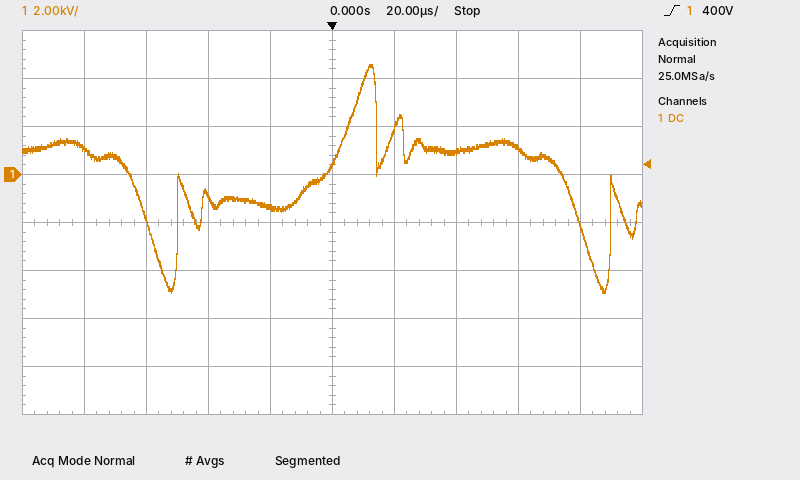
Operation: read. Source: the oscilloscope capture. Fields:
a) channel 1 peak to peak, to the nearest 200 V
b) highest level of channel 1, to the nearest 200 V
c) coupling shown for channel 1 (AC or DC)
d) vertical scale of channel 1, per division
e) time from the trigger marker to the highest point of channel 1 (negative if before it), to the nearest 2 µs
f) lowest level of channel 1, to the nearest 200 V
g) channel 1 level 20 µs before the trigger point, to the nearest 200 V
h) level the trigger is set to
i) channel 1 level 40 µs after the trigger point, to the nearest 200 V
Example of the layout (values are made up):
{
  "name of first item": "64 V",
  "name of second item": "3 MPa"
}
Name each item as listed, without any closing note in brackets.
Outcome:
{
  "channel 1 peak to peak, to the nearest 200 V": "9.6 kV",
  "highest level of channel 1, to the nearest 200 V": "4.6 kV",
  "coupling shown for channel 1": "DC",
  "vertical scale of channel 1, per division": "2 kV",
  "time from the trigger marker to the highest point of channel 1 (negative if before it), to the nearest 2 µs": "+12 µs",
  "lowest level of channel 1, to the nearest 200 V": "-5.0 kV",
  "channel 1 level 20 µs before the trigger point, to the nearest 200 V": "-1.4 kV",
  "level the trigger is set to": "400 V",
  "channel 1 level 40 µs after the trigger point, to the nearest 200 V": "1.0 kV"
}
